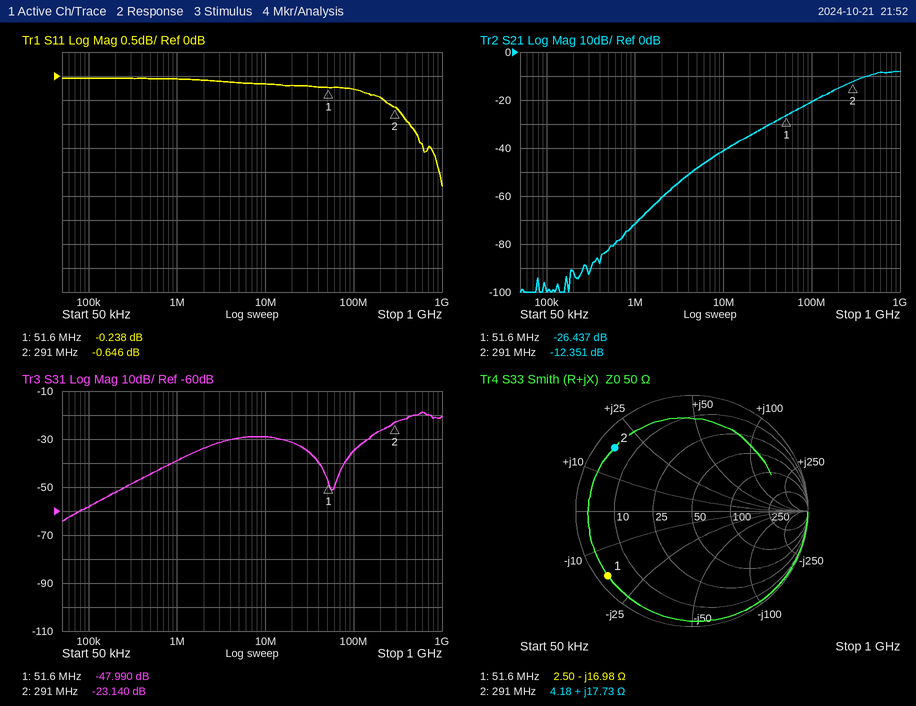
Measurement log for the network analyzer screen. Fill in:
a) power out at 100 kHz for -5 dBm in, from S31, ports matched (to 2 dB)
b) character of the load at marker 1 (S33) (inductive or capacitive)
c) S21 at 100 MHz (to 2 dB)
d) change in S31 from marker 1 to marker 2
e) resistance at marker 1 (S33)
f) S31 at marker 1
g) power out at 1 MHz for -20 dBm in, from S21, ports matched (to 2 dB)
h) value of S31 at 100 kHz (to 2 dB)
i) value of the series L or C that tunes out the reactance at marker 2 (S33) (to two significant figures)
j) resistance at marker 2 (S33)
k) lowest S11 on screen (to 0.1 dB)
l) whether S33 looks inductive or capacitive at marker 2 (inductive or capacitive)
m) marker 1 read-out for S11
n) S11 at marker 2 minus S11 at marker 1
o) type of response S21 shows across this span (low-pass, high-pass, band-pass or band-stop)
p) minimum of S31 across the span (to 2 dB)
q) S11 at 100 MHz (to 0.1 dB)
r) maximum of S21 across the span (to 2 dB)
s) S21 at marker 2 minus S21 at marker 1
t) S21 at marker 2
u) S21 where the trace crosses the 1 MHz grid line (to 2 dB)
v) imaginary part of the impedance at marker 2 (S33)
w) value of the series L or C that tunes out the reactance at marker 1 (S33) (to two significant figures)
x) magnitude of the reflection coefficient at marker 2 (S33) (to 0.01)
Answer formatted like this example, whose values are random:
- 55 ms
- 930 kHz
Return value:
- -64 dBm
- capacitive
- -20 dB
- 24.850 dB
- 2.50 Ω
- -47.990 dB
- -92 dBm
- -58 dB
- 31 pF
- 4.18 Ω
- -2.3 dB
- inductive
- -0.238 dB
- -0.408 dB
- high-pass
- -64 dB
- -0.3 dB
- -8 dB
- 14.086 dB
- -12.351 dB
- -72 dB
- +17.73 Ω
- 52 nH
- 0.86
